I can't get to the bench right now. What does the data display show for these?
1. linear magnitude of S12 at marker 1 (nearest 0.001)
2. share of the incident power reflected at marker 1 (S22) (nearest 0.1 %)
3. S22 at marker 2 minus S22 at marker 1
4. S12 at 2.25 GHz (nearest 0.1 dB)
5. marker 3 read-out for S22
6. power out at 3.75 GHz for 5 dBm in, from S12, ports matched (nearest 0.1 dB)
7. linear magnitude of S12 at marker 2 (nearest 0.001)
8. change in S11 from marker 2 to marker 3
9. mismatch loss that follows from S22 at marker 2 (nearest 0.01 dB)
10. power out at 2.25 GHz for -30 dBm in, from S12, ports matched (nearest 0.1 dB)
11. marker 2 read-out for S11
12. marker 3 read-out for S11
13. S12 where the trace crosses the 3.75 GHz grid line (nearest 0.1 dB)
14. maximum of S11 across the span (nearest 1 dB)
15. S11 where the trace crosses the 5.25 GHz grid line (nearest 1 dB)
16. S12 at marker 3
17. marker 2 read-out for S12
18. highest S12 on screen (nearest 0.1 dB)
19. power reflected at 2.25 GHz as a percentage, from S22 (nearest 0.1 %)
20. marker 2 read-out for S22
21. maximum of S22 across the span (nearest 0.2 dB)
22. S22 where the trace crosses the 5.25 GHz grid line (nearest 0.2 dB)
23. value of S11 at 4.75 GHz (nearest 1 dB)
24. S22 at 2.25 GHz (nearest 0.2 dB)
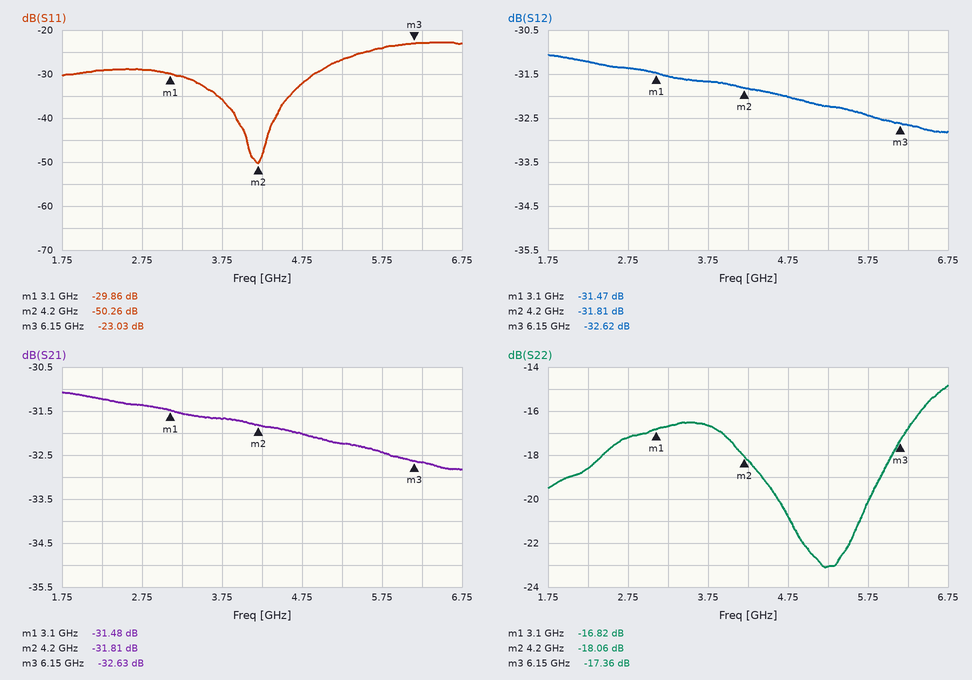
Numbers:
0.027
2.1 %
-1.24 dB
-31.2 dB
-17.36 dB
-26.7 dBm
0.026
27.23 dB
0.07 dB
-61.2 dBm
-50.26 dB
-23.03 dB
-31.7 dB
-23 dB
-27 dB
-32.62 dB
-31.81 dB
-31.1 dB
1.4 %
-18.06 dB
-14.8 dB
-23.0 dB
-32 dB
-18.6 dB
